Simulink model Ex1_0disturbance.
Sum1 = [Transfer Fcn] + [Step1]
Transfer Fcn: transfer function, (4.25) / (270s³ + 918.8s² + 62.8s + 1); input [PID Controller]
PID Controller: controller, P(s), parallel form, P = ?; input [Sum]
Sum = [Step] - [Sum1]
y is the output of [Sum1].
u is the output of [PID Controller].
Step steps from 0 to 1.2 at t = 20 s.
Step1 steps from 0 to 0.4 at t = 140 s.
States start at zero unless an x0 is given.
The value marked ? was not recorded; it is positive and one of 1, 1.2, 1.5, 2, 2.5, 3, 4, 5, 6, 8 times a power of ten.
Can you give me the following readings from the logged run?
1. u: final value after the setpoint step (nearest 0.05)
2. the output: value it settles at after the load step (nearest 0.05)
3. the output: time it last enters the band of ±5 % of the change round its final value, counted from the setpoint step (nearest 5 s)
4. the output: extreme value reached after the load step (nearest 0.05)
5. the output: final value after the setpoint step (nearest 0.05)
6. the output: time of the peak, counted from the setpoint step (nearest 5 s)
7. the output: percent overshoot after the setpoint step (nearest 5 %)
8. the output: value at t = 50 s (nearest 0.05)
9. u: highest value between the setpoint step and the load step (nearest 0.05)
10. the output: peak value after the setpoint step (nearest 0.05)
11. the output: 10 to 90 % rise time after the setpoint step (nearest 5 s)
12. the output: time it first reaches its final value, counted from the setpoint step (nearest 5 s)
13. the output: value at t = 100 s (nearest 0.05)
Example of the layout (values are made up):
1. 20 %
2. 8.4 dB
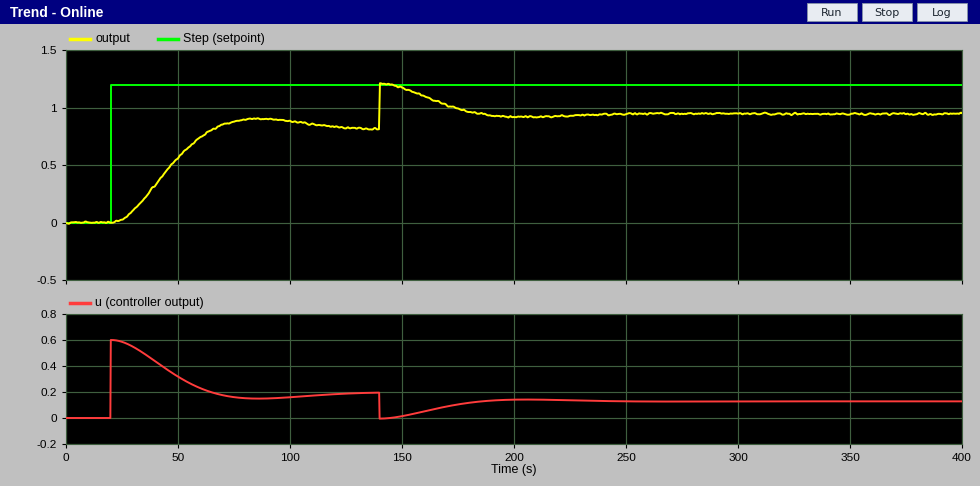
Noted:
1. 0.20
2. 0.95
3. 90 s
4. 1.20
5. 0.80
6. 65 s
7. 10 %
8. 0.55
9. 0.60
10. 0.90
11. 30 s
12. 45 s
13. 0.90
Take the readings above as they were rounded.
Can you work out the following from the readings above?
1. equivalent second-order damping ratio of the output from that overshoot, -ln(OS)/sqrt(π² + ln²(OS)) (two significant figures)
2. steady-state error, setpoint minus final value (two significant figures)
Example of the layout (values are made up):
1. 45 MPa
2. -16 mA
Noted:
1. 0.59
2. 0.40
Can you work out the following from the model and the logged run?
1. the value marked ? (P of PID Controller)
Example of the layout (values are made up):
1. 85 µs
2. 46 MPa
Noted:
1. 0.5
